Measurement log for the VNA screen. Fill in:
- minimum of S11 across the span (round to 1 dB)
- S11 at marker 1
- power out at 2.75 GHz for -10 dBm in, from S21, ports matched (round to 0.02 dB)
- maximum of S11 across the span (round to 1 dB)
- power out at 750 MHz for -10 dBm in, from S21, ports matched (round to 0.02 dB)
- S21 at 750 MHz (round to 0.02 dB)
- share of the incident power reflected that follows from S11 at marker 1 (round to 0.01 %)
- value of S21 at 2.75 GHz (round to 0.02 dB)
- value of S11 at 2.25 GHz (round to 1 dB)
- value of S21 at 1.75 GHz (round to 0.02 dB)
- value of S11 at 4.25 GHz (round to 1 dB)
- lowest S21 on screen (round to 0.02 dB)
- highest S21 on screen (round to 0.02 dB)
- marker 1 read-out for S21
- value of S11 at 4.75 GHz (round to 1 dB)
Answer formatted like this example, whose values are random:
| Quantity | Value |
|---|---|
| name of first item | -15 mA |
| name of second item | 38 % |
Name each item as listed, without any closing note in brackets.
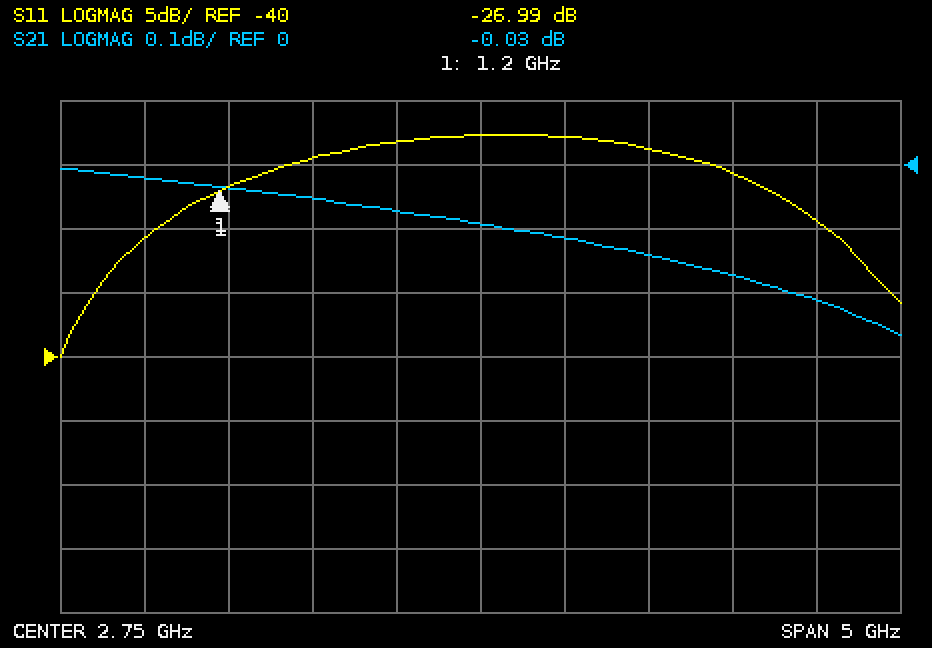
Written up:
| Quantity | Value |
|---|---|
| minimum of S11 across the span | -40 dB |
| S11 at marker 1 | -26.99 dB |
| power out at 2.75 GHz for -10 dBm in, from S21, ports matched | -10.10 dBm |
| maximum of S11 across the span | -23 dB |
| power out at 750 MHz for -10 dBm in, from S21, ports matched | -10.02 dBm |
| S21 at 750 MHz | -0.02 dB |
| share of the incident power reflected that follows from S11 at marker 1 | 0.20 % |
| value of S21 at 2.75 GHz | -0.10 dB |
| value of S11 at 2.25 GHz | -23 dB |
| value of S21 at 1.75 GHz | -0.06 dB |
| value of S11 at 4.25 GHz | -26 dB |
| lowest S21 on screen | -0.26 dB |
| highest S21 on screen | 0.00 dB |
| marker 1 read-out for S21 | -0.03 dB |
| value of S11 at 4.75 GHz | -29 dB |
